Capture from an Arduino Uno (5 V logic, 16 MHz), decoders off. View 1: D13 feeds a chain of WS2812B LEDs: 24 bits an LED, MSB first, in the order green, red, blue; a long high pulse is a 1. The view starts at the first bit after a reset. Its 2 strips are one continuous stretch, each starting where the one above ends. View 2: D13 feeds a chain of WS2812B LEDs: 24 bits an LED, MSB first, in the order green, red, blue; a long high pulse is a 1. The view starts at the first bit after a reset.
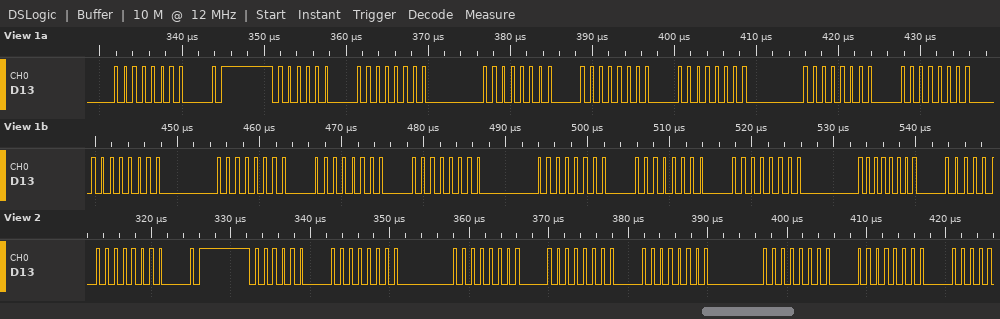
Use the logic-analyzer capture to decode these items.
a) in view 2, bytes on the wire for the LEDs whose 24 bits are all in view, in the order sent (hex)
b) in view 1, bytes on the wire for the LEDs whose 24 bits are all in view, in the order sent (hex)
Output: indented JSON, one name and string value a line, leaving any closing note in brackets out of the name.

{
  "in view 2, bytes on the wire for the LEDs whose 24 bits are all in view, in the order sent": "00 40 00 00 00 00",
  "in view 1, bytes on the wire for the LEDs whose 24 bits are all in view, in the order sent": "00 40 00 00 00 00 00 00 00 00 00 00 00 00 00"
}
